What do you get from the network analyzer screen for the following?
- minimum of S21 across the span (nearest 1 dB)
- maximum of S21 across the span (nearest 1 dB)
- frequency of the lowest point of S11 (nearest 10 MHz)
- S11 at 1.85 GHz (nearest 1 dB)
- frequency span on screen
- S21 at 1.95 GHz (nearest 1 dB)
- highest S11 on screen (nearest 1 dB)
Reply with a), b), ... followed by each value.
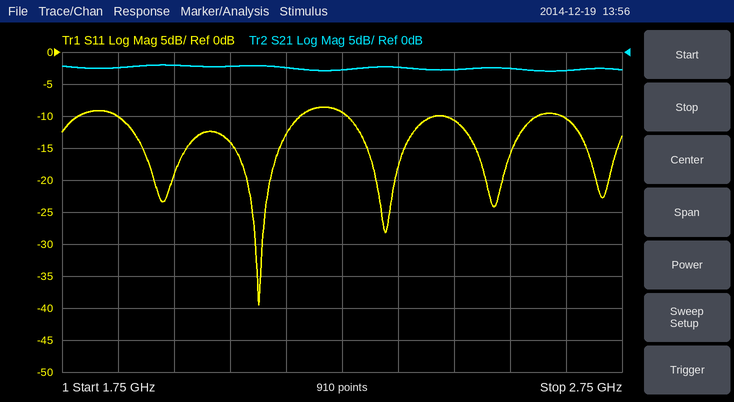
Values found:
a) -3 dB
b) -2 dB
c) 2.10 GHz
d) -10 dB
e) 1 GHz
f) -2 dB
g) -9 dB
